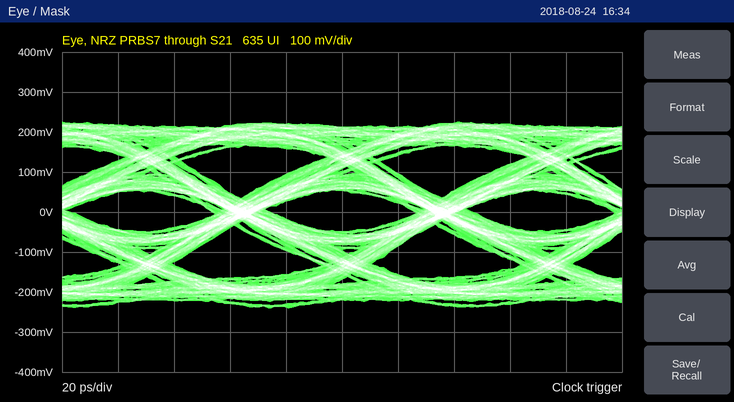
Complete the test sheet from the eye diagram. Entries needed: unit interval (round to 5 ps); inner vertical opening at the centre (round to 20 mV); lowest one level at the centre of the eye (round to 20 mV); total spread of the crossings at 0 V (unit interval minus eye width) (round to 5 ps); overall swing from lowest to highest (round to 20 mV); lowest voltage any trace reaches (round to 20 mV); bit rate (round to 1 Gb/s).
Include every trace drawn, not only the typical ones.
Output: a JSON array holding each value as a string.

["70 ps", "100 mV", "60 mV", "20 ps", "460 mV", "-240 mV", "14 Gb/s"]
